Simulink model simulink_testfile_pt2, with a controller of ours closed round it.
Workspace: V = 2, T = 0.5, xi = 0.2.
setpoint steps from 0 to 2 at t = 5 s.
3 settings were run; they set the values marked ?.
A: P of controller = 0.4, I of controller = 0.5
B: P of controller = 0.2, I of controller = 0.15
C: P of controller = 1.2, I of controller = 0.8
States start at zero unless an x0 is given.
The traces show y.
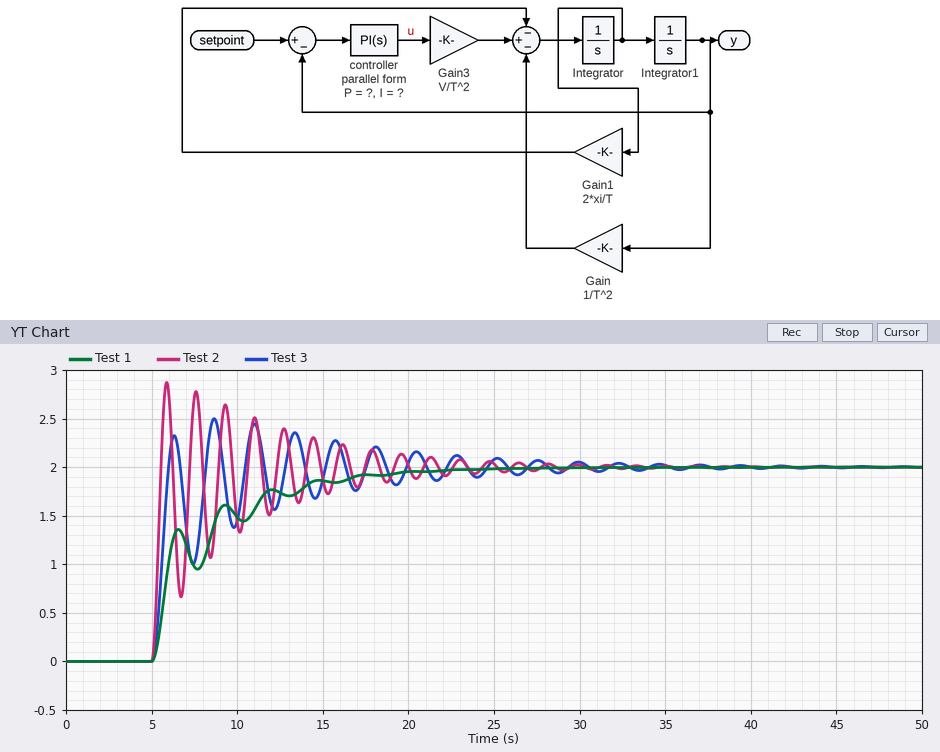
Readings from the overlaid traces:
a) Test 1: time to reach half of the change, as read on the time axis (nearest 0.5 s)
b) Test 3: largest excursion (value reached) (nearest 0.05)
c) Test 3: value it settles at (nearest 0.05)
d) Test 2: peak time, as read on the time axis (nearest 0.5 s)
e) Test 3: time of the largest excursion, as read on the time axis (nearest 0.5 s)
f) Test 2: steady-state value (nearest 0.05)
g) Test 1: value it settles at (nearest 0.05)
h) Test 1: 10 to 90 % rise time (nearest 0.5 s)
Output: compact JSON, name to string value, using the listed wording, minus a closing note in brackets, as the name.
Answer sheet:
{"Test 1: time to reach half of the change, as read on the time axis": "6.0 s", "Test 3: largest excursion (value reached)": "2.50", "Test 3: value it settles at": "2.00", "Test 2: peak time, as read on the time axis": "6.0 s", "Test 3: time of the largest excursion, as read on the time axis": "8.5 s", "Test 2: steady-state value": "2.00", "Test 1: value it settles at": "2.00", "Test 1: 10 to 90 % rise time": "8.5 s"}
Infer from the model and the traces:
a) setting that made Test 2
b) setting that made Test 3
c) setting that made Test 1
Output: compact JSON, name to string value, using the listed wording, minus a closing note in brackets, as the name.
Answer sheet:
{"setting that made Test 2": "C", "setting that made Test 3": "A", "setting that made Test 1": "B"}
